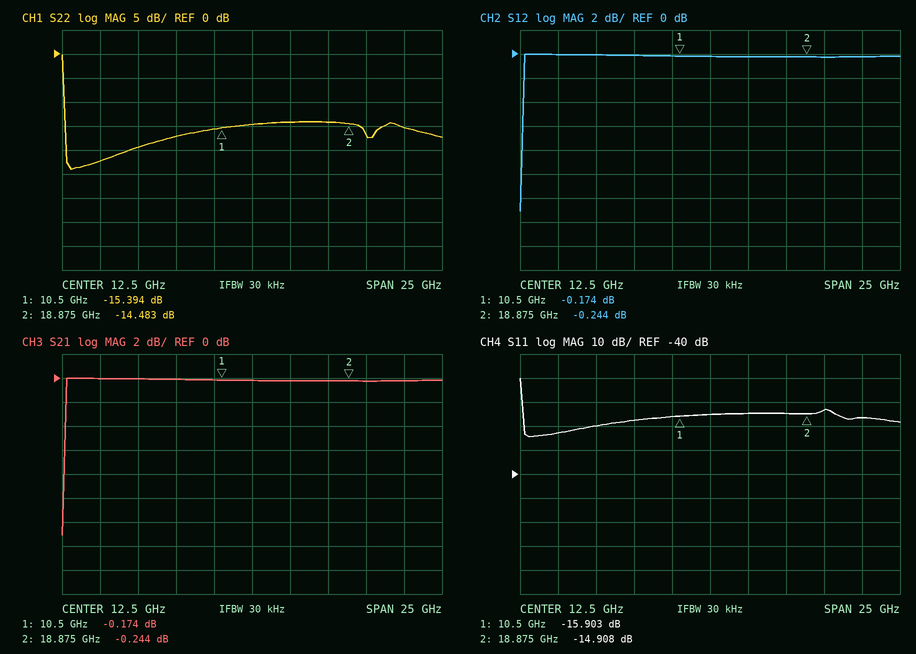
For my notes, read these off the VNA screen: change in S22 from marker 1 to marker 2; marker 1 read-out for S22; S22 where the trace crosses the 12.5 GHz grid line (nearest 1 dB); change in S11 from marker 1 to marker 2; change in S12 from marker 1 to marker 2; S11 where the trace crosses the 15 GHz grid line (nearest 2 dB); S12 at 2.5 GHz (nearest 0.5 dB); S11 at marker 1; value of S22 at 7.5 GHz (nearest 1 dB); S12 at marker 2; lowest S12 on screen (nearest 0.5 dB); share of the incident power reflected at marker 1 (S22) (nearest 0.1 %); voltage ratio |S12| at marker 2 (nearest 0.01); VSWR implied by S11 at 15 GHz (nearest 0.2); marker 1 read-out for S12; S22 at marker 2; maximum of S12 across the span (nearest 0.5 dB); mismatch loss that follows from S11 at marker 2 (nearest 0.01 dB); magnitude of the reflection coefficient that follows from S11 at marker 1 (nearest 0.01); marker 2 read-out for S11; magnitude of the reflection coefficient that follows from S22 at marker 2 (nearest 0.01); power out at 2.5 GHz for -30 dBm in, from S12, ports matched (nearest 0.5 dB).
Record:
0.911 dB
-15.394 dB
-15 dB
0.995 dB
-0.070 dB
-14 dB
0.0 dB
-15.903 dB
-17 dB
-0.244 dB
-13.0 dB
2.9 %
0.97
1.4
-0.174 dB
-14.483 dB
0.0 dB
0.14 dB
0.16
-14.908 dB
0.19
-30.0 dBm
